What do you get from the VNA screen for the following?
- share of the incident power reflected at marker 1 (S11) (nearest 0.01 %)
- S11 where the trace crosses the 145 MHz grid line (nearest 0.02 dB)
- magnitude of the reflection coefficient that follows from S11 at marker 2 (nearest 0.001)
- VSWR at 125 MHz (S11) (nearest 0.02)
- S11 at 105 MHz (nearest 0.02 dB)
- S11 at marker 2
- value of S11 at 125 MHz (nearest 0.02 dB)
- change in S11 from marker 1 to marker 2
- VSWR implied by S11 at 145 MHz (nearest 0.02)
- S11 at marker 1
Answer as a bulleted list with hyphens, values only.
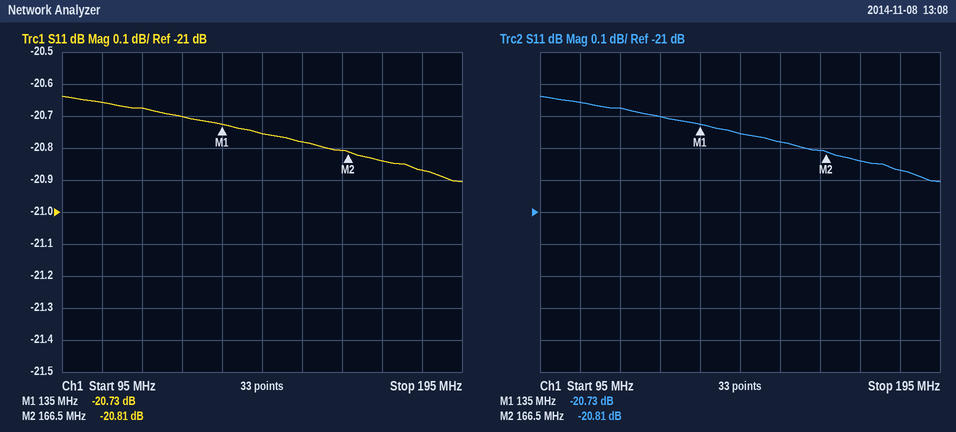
- 0.85 %
- -20.76 dB
- 0.091
- 1.20
- -20.66 dB
- -20.81 dB
- -20.70 dB
- -0.08 dB
- 1.20
- -20.73 dB
